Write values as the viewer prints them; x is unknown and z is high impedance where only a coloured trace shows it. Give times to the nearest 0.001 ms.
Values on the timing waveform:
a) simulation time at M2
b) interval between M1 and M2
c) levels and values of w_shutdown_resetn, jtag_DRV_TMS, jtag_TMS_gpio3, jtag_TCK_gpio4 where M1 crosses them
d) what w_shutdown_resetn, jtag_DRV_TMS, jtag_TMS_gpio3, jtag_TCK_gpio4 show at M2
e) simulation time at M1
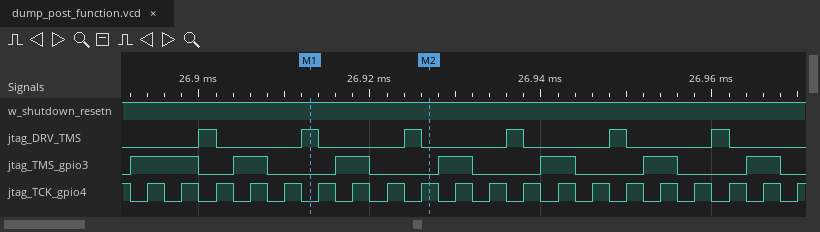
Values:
26.927 ms
0.014 ms
w_shutdown_resetn=1, jtag_DRV_TMS=1, jtag_TMS_gpio3=0, jtag_TCK_gpio4=0
w_shutdown_resetn=1, jtag_DRV_TMS=0, jtag_TMS_gpio3=0, jtag_TCK_gpio4=1
26.913 ms
